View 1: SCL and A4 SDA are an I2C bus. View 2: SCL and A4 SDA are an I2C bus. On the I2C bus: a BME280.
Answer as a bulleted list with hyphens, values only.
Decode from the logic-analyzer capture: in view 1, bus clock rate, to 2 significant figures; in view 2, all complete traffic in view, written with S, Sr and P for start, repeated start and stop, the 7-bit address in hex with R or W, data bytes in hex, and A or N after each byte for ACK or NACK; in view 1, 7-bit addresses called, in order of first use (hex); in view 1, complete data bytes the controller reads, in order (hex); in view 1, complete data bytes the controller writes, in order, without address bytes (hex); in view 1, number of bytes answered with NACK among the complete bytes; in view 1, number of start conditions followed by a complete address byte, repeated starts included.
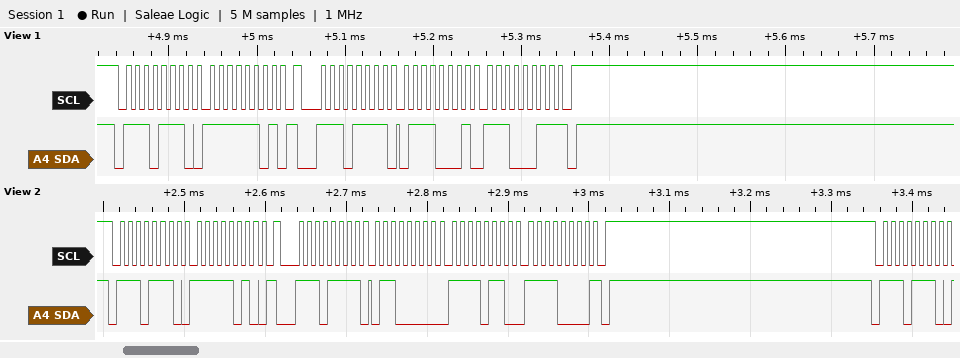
- 100 kHz
- S 77W A FA A Sr 77R A 60 A F6 A F0 N P S 77W A
- 0x77
- 71 E3
- FD
- 1
- 2
